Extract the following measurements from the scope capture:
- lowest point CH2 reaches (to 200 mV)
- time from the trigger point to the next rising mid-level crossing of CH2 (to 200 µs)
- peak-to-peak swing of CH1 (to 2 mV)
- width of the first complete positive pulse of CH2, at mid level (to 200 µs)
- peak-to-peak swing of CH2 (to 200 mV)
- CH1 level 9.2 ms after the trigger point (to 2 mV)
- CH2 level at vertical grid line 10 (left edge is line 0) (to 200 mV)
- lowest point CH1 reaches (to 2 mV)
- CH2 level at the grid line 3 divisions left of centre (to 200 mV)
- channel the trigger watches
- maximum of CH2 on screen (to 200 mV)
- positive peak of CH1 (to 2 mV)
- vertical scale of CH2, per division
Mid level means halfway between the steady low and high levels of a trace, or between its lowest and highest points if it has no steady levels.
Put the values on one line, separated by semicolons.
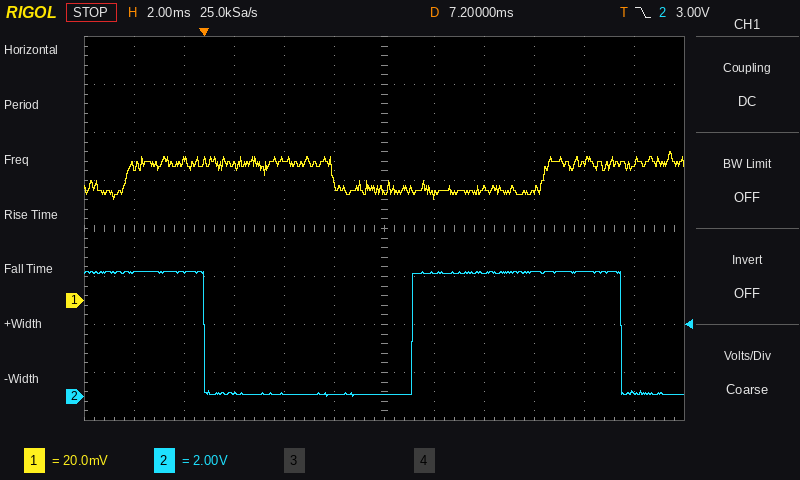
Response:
0.0 V; 8.4 ms; 20 mV; 8.4 ms; 5.2 V; 44 mV; 5.2 V; 42 mV; 200 mV; CH2; 5.2 V; 62 mV; 2 V
